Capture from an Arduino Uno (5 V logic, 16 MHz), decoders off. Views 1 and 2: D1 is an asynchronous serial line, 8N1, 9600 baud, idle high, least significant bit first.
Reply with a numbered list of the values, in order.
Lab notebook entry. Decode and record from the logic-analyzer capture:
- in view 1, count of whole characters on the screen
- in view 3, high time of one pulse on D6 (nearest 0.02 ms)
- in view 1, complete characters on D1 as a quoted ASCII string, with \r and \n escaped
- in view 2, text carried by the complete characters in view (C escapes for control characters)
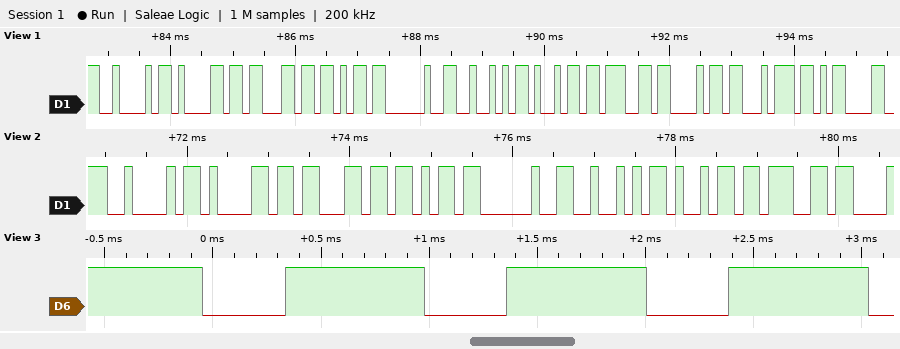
1. 11
2. 0.64 ms
3. "Back Right\r"
4. "Back Rig"
